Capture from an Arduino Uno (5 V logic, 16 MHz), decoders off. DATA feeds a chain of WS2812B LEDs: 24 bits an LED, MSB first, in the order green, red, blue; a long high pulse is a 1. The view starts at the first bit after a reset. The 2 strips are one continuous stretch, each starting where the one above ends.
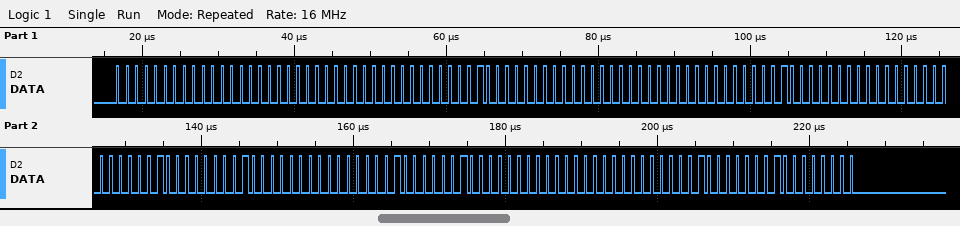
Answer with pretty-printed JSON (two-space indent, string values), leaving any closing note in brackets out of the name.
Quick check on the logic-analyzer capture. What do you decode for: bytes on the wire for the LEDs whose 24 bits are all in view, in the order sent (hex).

{
  "bytes on the wire for the LEDs whose 24 bits are all in view, in the order sent": "00 00 00 00 02 00 00 00 02 00 00 02 01 00 01 02 00 00 01 01 00"
}
